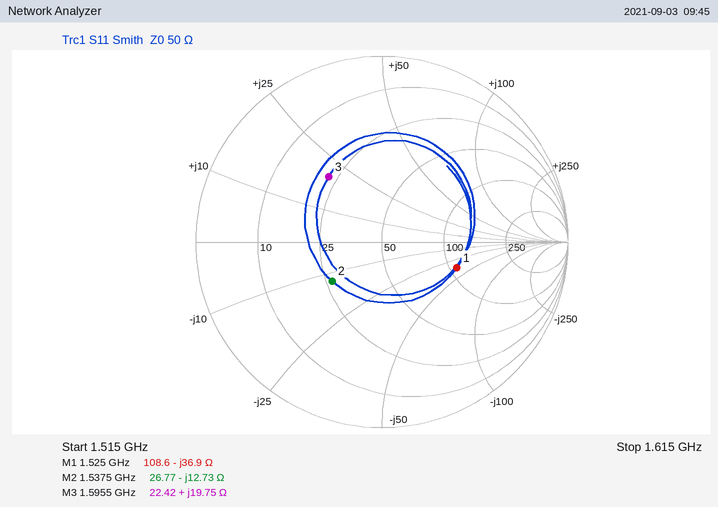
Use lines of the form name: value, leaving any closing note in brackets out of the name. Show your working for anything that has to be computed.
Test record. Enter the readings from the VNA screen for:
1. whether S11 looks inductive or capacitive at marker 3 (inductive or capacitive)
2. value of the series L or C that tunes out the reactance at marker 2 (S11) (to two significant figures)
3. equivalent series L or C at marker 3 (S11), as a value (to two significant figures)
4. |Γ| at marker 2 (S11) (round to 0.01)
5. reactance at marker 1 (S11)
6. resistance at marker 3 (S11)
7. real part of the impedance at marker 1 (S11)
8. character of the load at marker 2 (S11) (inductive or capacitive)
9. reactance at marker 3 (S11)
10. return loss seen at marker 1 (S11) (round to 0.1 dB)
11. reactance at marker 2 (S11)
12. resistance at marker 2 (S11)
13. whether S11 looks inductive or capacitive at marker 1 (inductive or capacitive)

whether S11 looks inductive or capacitive at marker 3: inductive
value of the series L or C that tunes out the reactance at marker 2 (S11): L = 12.73 Ω/(2π × 1.5375 GHz) ≈ 1.3 nH
equivalent series L or C at marker 3 (S11), as a value: L = 19.75 Ω/(2π × 1.5955 GHz) ≈ 2.0 nH
|Γ| at marker 2 (S11): 0.34
reactance at marker 1: -36.9 Ω
resistance at marker 3: 22.42 Ω
real part of the impedance at marker 1: 108.6 Ω
character of the load at marker 2 (S11): capacitive
reactance at marker 3: +19.75 Ω
return loss seen at marker 1 (S11): 7.4 dB
reactance at marker 2: -12.73 Ω
resistance at marker 2: 26.77 Ω
whether S11 looks inductive or capacitive at marker 1: capacitive
